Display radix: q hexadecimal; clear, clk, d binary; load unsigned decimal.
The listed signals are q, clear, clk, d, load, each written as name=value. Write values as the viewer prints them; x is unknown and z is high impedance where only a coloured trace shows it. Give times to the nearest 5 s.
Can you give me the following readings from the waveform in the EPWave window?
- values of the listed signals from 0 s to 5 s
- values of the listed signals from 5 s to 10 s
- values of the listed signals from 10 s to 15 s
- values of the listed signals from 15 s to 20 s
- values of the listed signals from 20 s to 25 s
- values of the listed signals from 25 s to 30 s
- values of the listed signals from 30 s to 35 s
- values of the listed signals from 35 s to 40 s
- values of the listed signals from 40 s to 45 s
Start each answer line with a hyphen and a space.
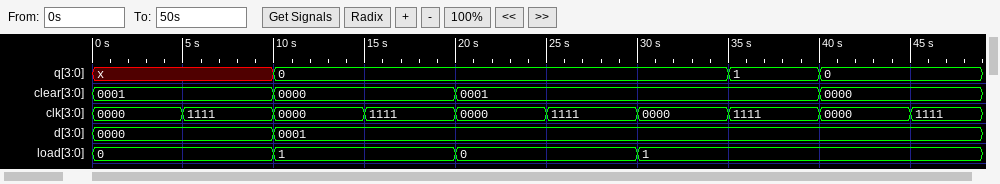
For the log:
- q=x, clear=0001, clk=0000, d=0000, load=0
- q=x, clear=0001, clk=1111, d=0000, load=0
- q=0, clear=0000, clk=0000, d=0001, load=1
- q=0, clear=0000, clk=1111, d=0001, load=1
- q=0, clear=0001, clk=0000, d=0001, load=0
- q=0, clear=0001, clk=1111, d=0001, load=0
- q=0, clear=0001, clk=0000, d=0001, load=1
- q=1, clear=0001, clk=1111, d=0001, load=1
- q=0, clear=0000, clk=0000, d=0001, load=1
